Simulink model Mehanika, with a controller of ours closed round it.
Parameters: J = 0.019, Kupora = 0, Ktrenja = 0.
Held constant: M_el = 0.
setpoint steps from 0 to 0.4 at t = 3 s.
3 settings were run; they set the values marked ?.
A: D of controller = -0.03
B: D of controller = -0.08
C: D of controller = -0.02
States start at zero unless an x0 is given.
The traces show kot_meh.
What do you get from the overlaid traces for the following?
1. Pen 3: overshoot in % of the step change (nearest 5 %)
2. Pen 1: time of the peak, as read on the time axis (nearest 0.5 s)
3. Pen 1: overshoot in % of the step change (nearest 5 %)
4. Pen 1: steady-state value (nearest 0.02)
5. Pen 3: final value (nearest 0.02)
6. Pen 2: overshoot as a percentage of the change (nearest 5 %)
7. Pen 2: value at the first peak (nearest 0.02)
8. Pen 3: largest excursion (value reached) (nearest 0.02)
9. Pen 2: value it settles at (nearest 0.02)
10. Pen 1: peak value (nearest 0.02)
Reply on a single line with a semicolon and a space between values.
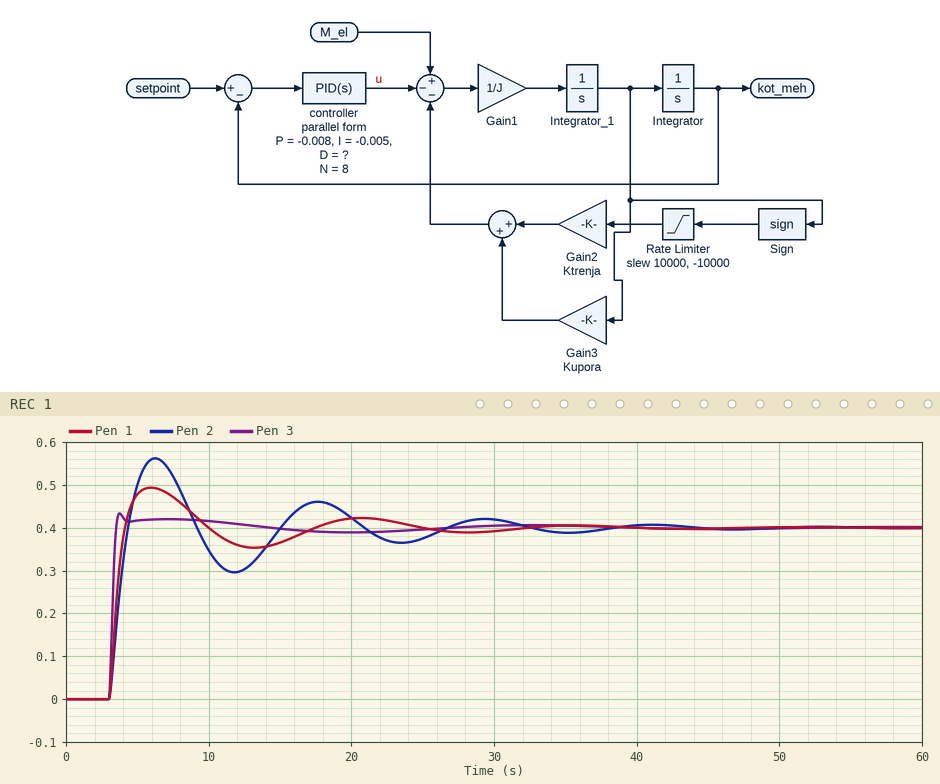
10 %; 6.0 s; 25 %; 0.40; 0.40; 40 %; 0.56; 0.44; 0.40; 0.50
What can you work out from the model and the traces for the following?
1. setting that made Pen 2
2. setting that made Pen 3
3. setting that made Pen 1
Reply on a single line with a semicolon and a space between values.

C; B; A
